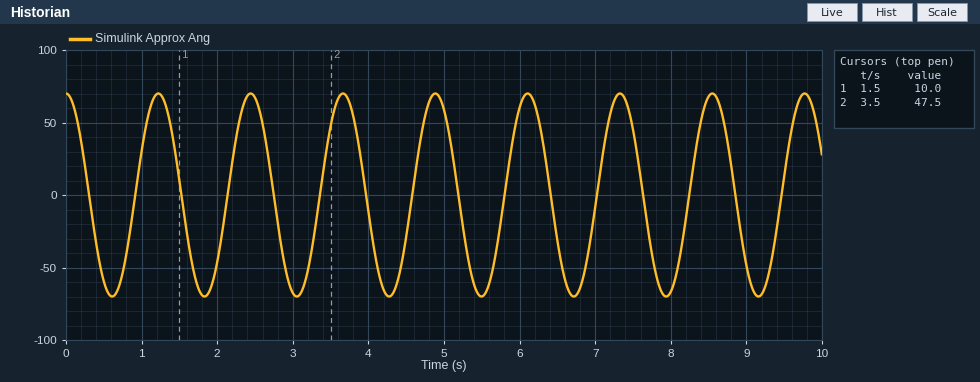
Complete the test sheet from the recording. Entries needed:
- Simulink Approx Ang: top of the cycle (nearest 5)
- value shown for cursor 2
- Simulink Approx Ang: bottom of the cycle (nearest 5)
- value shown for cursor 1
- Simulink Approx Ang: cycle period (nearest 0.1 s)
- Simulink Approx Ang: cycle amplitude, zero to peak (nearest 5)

70
47.5
-70
10.0
1.2 s
70
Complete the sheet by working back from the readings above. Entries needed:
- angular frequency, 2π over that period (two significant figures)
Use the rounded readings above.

5.2 rad/s
